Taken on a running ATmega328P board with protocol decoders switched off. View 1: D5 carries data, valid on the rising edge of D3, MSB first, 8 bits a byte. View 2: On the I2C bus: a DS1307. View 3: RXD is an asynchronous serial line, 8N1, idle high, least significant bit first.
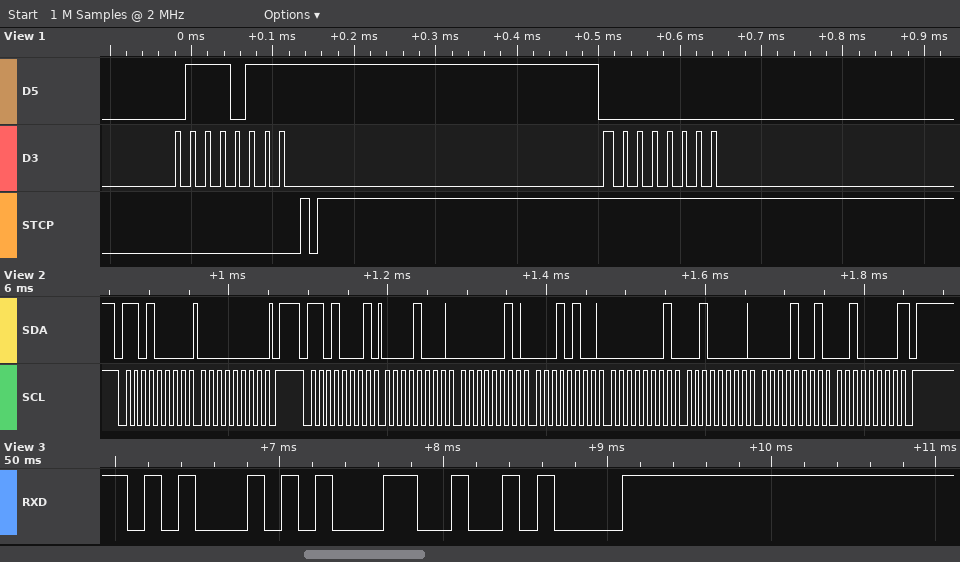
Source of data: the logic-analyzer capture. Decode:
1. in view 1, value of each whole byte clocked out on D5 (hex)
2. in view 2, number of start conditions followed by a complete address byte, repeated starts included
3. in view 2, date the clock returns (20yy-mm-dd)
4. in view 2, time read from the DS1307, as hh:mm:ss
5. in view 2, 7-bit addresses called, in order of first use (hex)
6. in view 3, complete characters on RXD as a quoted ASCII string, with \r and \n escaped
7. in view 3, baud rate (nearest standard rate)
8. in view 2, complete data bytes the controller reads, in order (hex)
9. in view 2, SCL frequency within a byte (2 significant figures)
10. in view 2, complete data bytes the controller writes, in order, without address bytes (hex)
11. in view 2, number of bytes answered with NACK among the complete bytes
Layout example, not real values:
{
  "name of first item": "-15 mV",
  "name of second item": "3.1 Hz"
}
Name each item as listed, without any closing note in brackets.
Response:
{
  "in view 1, value of each whole byte clocked out on D5": "77 00",
  "in view 2, number of start conditions followed by a complete address byte, repeated starts included": "2",
  "in view 2, date the clock returns": "2020-09-20",
  "in view 2, time read from the DS1307, as hh:mm:ss": "14:02:08",
  "in view 2, 7-bit addresses called, in order of first use": "0x68",
  "in view 3, complete characters on RXD as a quoted ASCII string, with \\r and \\n escaped": "\"E1\\n\"",
  "in view 3, baud rate": "9600 baud",
  "in view 2, complete data bytes the controller reads, in order": "08 02 14 01 20 09 20",
  "in view 2, SCL frequency within a byte": "100 kHz",
  "in view 2, complete data bytes the controller writes, in order, without address bytes": "00",
  "in view 2, number of bytes answered with NACK among the complete bytes": "1"
}
